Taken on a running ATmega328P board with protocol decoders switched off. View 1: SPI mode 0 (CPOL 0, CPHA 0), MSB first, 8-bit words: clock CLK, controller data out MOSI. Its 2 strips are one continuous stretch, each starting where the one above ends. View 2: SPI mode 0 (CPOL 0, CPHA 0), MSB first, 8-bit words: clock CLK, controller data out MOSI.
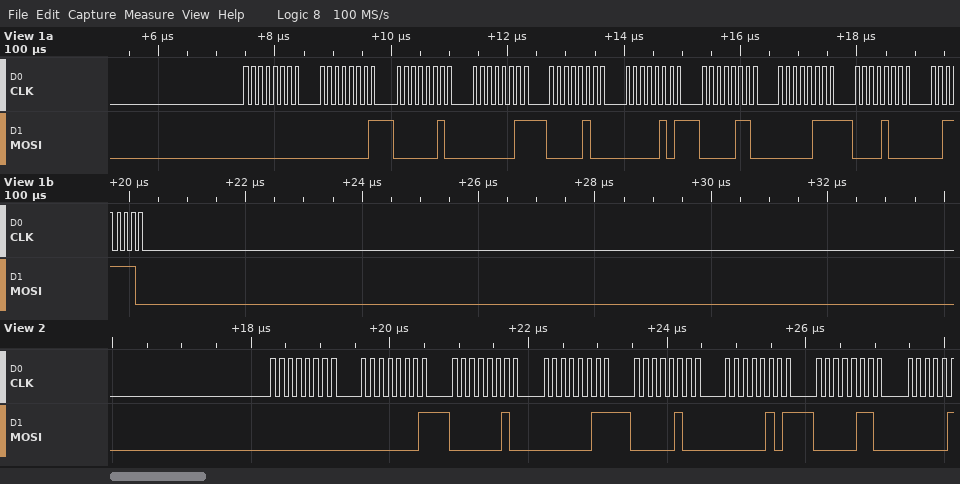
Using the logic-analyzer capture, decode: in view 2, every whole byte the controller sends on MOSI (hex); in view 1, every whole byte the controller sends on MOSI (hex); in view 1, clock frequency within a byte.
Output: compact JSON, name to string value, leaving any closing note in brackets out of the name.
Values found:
{"in view 2, every whole byte the controller sends on MOSI": "00 01 02 03 04 05 06", "in view 1, every whole byte the controller sends on MOSI": "0x00 0x01 0x02 0x03 0x04 0x05 0x06 0x07 0x08 0x3E", "in view 1, clock frequency within a byte": "8 MHz"}
